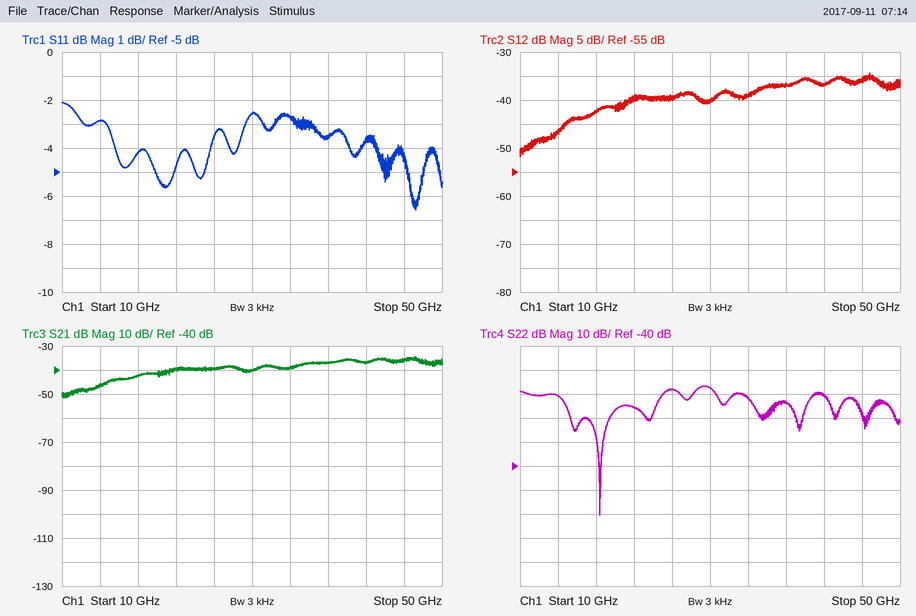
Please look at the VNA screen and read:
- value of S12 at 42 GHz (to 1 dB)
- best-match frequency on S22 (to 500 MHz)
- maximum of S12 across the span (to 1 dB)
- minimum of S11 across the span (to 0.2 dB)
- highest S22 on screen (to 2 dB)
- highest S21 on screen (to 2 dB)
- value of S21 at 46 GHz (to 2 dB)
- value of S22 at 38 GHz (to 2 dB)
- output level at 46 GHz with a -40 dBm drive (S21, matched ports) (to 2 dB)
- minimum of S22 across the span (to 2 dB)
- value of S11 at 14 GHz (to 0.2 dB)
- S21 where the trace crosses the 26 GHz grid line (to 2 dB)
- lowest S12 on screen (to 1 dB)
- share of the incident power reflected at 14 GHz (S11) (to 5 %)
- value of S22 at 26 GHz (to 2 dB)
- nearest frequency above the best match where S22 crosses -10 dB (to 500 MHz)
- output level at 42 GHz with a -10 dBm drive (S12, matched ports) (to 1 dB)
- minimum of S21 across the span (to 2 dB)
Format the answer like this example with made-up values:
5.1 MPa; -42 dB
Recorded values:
-37 dB; 18.5 GHz; -34 dB; -6.6 dB; -6 dB; -34 dB; -36 dB; -14 dB; -76 dBm; -60 dB; -2.8 dB; -40 dB; -52 dB; 50 %; -8 dB; 25.0 GHz; -47 dBm; -52 dB
